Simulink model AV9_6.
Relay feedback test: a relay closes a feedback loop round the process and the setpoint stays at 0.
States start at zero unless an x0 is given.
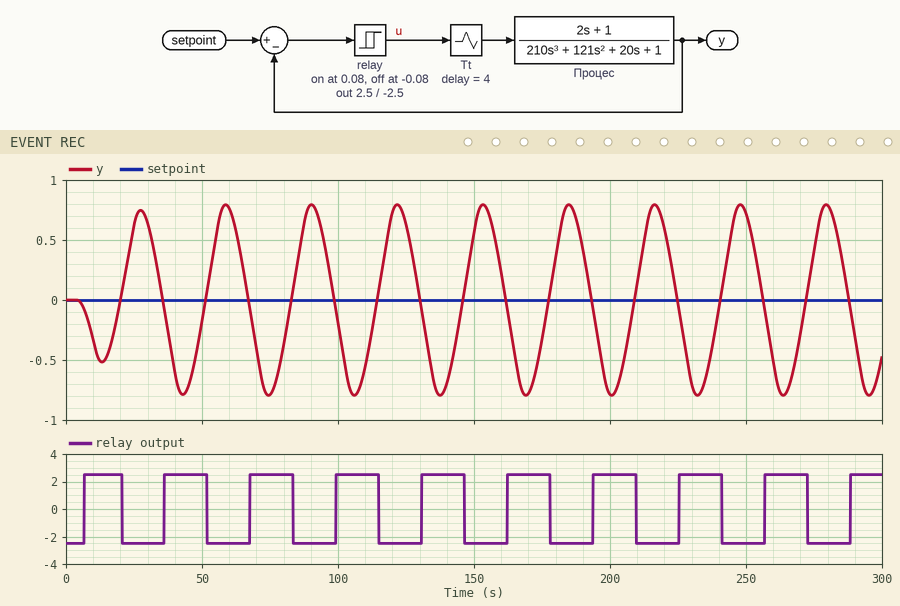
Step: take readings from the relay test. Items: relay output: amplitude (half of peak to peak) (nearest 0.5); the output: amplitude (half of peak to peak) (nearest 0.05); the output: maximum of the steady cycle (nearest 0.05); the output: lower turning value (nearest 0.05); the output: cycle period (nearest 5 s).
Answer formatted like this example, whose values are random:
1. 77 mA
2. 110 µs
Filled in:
1. 2.5
2. 0.80
3. 0.80
4. -0.80
5. 30 s
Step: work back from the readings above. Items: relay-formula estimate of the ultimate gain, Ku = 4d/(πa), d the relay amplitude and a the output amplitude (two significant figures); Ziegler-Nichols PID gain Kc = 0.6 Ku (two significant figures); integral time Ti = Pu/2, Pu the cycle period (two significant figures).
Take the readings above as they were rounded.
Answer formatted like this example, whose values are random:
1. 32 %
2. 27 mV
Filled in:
1. 4.0
2. 2.4
3. 15 s
